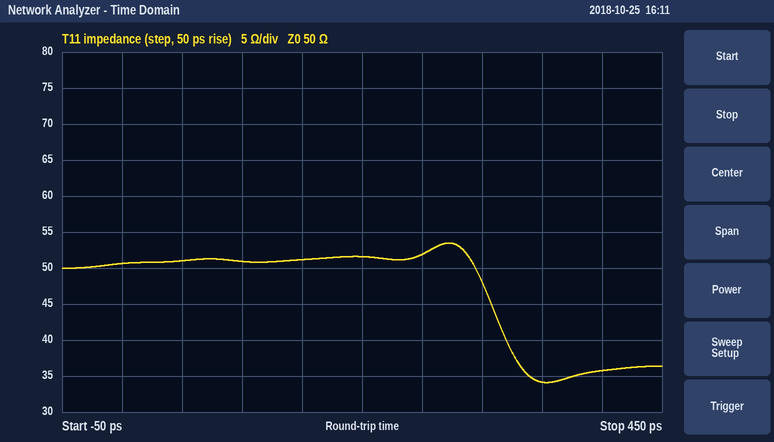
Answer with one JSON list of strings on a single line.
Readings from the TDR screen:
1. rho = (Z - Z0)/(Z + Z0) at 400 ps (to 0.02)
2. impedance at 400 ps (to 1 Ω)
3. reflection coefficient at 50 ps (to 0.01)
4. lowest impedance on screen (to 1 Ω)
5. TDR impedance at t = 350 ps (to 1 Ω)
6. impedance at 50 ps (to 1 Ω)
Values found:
["-0.16", "36 Ω", "+0.01", "34 Ω", "34 Ω", "51 Ω"]
